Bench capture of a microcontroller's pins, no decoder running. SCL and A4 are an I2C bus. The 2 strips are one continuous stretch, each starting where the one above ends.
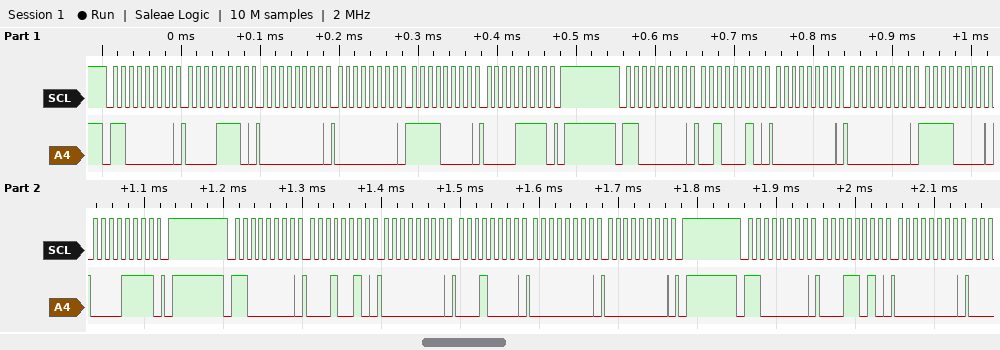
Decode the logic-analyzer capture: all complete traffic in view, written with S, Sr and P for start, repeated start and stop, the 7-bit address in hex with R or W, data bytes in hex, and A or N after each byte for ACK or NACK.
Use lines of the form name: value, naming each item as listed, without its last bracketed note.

all complete traffic in view, written with S, Sr and P for start, repeated start and stop, the 7-bit address in hex with R or W, data bytes in hex, and A or N after each byte for ACK or NACK: S 60W A 0E A 00 A 00 A F0 A 0F A P S 60W A 22 A 00 A 00 A F0 A 0F A P S 60W A 12 A 00 A 10 A 00 A 00 A P S 60W A 1A A 00 A
